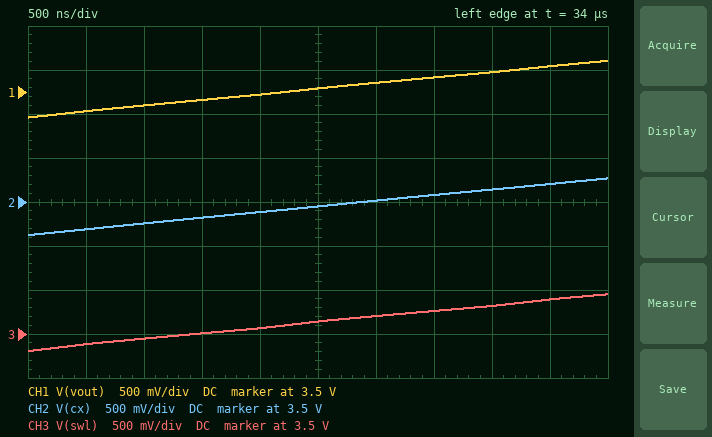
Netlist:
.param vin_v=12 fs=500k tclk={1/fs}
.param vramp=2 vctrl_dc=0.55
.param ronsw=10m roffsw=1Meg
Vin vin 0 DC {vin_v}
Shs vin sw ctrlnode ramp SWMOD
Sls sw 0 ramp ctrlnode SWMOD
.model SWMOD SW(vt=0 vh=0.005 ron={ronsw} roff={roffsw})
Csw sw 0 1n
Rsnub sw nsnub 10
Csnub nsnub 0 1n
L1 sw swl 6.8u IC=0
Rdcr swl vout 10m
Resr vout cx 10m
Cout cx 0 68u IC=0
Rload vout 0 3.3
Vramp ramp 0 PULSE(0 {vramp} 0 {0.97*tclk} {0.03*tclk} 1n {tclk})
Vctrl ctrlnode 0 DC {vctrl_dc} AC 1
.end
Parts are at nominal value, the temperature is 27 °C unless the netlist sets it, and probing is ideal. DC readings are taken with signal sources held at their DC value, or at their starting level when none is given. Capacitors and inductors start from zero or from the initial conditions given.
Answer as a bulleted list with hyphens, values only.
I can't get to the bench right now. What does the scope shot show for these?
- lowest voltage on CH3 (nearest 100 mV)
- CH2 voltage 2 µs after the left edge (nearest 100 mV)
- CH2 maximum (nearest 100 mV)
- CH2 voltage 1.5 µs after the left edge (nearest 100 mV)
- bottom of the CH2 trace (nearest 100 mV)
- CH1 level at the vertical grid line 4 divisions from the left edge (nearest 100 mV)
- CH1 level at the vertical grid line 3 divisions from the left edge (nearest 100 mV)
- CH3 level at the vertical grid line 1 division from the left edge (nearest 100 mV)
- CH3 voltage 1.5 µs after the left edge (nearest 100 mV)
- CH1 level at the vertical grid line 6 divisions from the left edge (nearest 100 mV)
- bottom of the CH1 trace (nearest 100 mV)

- 3.3 V
- 3.4 V
- 3.8 V
- 3.3 V
- 3.1 V
- 3.5 V
- 3.4 V
- 3.4 V
- 3.5 V
- 3.6 V
- 3.2 V
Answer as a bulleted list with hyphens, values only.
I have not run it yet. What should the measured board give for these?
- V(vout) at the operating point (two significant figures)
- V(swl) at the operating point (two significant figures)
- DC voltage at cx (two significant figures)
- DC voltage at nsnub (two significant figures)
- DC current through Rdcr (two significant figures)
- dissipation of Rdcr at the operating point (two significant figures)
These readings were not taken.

- 12 V
- 12 V
- 12 V
- 12 V
- 3.6 A
- 130 mW
